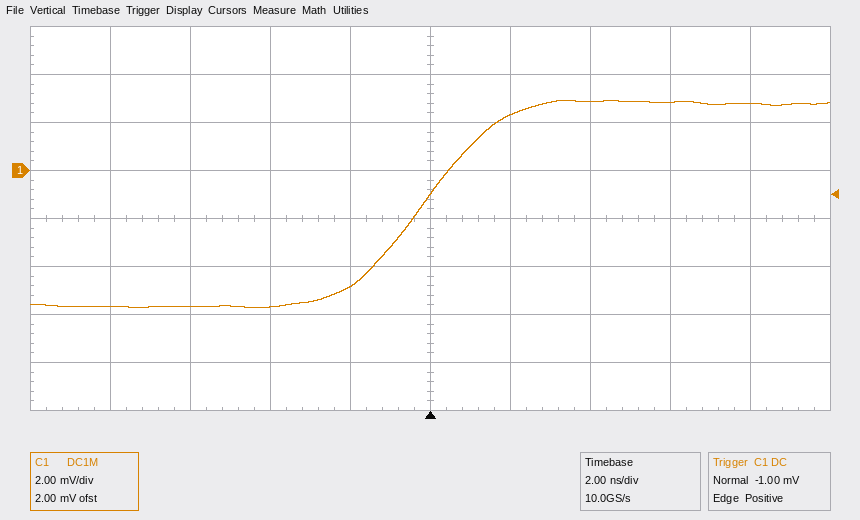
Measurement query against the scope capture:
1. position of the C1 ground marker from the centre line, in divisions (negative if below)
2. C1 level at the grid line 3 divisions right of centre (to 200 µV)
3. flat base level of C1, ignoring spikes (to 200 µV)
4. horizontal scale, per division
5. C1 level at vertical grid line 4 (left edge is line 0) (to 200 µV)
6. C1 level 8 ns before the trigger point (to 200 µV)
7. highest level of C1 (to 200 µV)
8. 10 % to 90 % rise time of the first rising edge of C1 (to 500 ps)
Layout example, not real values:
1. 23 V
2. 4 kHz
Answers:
1. +1.0 div
2. 2.8 mV
3. -5.6 mV
4. 2 ns
5. -4.8 mV
6. -5.6 mV
7. 3.0 mV
8. 3.5 ns
